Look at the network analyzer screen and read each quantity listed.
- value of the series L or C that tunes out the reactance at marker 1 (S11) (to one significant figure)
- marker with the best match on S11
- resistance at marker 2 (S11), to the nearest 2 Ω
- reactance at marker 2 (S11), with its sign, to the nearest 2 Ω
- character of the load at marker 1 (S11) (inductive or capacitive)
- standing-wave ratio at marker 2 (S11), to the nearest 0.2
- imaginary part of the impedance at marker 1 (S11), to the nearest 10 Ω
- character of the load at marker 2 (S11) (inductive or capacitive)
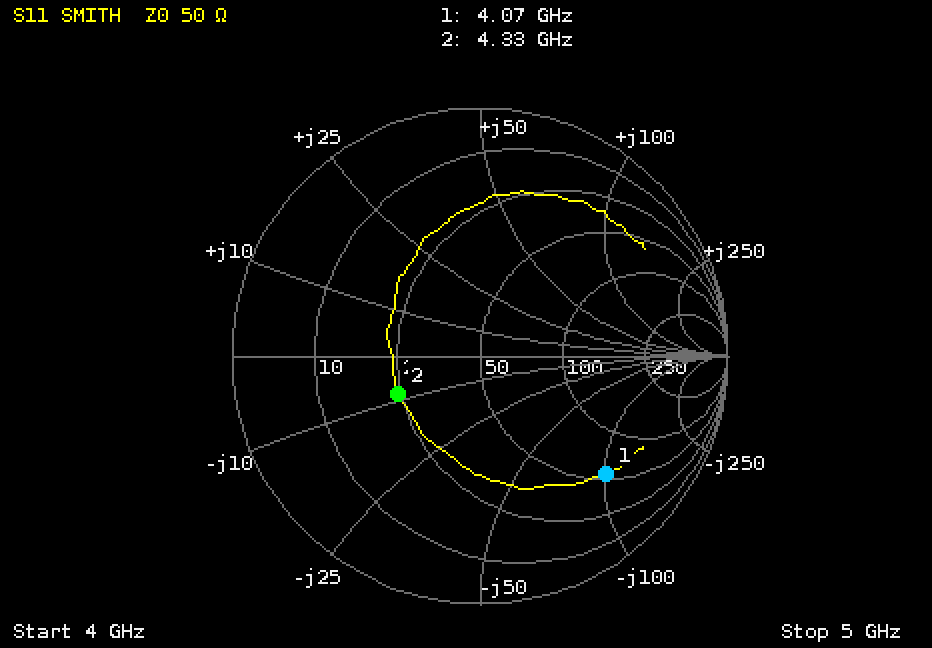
4 nH
marker 2
24 Ω
-8 Ω
capacitive
2.2
-100 Ω
capacitive
